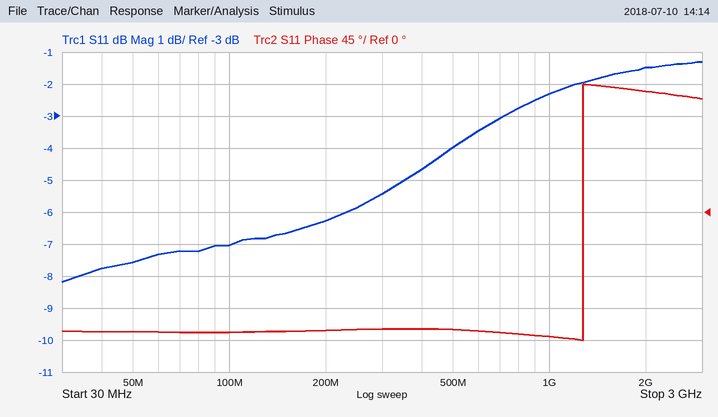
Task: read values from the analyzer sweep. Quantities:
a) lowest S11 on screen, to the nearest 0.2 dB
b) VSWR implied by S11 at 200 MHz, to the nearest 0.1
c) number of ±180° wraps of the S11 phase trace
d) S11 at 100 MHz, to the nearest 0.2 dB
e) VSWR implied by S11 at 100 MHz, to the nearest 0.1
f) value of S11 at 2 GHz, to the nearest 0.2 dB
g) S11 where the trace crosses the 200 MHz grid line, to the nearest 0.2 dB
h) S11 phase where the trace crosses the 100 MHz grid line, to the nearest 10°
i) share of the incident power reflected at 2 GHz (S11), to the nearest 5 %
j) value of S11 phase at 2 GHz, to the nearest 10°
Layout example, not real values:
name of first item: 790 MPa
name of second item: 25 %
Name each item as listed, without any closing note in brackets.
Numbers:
lowest S11 on screen, to the nearest 0.2 dB: -8.2 dB
VSWR implied by S11 at 200 MHz, to the nearest 0.1: 2.9
number of ±180° wraps of the S11 phase trace: 1
S11 at 100 MHz, to the nearest 0.2 dB: -7.0 dB
VSWR implied by S11 at 100 MHz, to the nearest 0.1: 2.6
value of S11 at 2 GHz, to the nearest 0.2 dB: -1.4 dB
S11 where the trace crosses the 200 MHz grid line, to the nearest 0.2 dB: -6.2 dB
S11 phase where the trace crosses the 100 MHz grid line, to the nearest 10°: -170°
share of the incident power reflected at 2 GHz (S11), to the nearest 5 %: 70 %
value of S11 phase at 2 GHz, to the nearest 10°: 170°
